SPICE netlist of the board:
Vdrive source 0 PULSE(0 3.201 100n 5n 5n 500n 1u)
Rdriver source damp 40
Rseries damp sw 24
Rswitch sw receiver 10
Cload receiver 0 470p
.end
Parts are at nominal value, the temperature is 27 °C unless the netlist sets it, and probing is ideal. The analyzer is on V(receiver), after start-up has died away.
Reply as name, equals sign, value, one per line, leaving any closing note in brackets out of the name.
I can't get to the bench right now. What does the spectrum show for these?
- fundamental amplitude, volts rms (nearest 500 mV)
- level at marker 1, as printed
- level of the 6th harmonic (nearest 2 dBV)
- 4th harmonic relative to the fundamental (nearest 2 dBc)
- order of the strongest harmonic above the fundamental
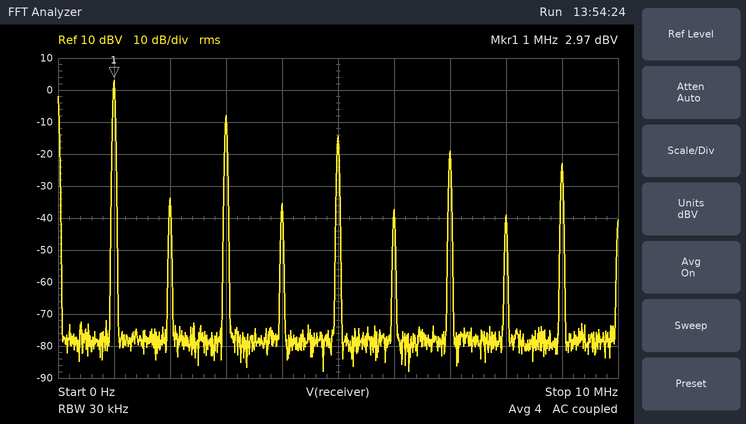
fundamental amplitude, volts rms = 1.5 V
level at marker 1, as printed = 2.97 dBV
level of the 6th harmonic = -38 dBV
4th harmonic relative to the fundamental = -38 dBc
order of the strongest harmonic above the fundamental = 3
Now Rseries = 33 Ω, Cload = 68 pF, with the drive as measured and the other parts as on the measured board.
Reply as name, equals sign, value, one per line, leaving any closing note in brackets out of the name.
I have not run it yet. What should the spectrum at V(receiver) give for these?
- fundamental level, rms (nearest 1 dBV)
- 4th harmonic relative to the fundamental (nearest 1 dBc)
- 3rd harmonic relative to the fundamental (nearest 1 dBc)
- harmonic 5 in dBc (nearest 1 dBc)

fundamental level, rms = 3 dBV
4th harmonic relative to the fundamental = -36 dBc
3rd harmonic relative to the fundamental = -10 dBc
harmonic 5 in dBc = -14 dBc
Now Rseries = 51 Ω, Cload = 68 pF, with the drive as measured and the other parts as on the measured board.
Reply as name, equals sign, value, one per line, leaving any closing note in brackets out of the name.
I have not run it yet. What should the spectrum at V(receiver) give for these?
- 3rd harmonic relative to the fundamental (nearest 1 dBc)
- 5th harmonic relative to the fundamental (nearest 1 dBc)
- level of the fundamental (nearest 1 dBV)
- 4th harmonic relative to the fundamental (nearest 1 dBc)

3rd harmonic relative to the fundamental = -10 dBc
5th harmonic relative to the fundamental = -14 dBc
level of the fundamental = 3 dBV
4th harmonic relative to the fundamental = -36 dBc
